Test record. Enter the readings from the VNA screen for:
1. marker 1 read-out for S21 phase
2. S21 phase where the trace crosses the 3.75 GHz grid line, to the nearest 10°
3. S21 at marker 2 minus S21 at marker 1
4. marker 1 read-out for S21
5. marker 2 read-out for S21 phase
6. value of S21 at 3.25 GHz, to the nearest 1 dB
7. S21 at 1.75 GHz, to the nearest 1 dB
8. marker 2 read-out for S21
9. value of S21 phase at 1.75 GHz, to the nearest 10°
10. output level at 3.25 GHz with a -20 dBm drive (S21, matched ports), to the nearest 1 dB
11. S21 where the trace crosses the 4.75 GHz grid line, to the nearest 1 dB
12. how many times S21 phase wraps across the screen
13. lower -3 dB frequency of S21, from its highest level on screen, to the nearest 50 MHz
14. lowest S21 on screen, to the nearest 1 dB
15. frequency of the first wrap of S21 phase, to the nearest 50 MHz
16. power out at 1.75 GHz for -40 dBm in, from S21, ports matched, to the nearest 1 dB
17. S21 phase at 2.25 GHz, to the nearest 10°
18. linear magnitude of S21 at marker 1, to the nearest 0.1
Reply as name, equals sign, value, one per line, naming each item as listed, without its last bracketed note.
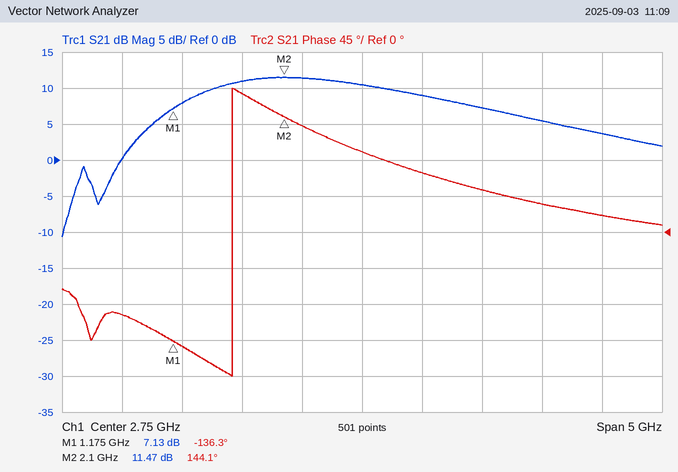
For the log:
marker 1 read-out for S21 phase = -136.3°
S21 phase where the trace crosses the 3.75 GHz grid line, to the nearest 10° = 50°
S21 at marker 2 minus S21 at marker 1 = 4.34 dB
marker 1 read-out for S21 = 7.13 dB
marker 2 read-out for S21 phase = 144.1°
value of S21 at 3.25 GHz, to the nearest 1 dB = 9 dB
S21 at 1.75 GHz, to the nearest 1 dB = 11 dB
marker 2 read-out for S21 = 11.47 dB
value of S21 phase at 1.75 GHz, to the nearest 10° = 170°
output level at 3.25 GHz with a -20 dBm drive (S21, matched ports), to the nearest 1 dB = -11 dBm
S21 where the trace crosses the 4.75 GHz grid line, to the nearest 1 dB = 4 dB
how many times S21 phase wraps across the screen = 1
lower -3 dB frequency of S21, from its highest level on screen, to the nearest 50 MHz = 1.30 GHz
lowest S21 on screen, to the nearest 1 dB = -11 dB
frequency of the first wrap of S21 phase, to the nearest 50 MHz = 1.65 GHz
power out at 1.75 GHz for -40 dBm in, from S21, ports matched, to the nearest 1 dB = -29 dBm
S21 phase at 2.25 GHz, to the nearest 10° = 130°
linear magnitude of S21 at marker 1, to the nearest 0.1 = 2.3
